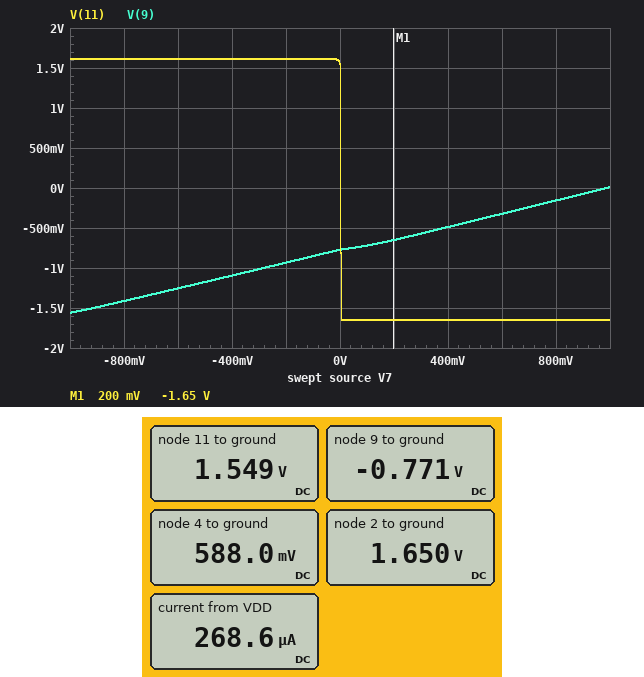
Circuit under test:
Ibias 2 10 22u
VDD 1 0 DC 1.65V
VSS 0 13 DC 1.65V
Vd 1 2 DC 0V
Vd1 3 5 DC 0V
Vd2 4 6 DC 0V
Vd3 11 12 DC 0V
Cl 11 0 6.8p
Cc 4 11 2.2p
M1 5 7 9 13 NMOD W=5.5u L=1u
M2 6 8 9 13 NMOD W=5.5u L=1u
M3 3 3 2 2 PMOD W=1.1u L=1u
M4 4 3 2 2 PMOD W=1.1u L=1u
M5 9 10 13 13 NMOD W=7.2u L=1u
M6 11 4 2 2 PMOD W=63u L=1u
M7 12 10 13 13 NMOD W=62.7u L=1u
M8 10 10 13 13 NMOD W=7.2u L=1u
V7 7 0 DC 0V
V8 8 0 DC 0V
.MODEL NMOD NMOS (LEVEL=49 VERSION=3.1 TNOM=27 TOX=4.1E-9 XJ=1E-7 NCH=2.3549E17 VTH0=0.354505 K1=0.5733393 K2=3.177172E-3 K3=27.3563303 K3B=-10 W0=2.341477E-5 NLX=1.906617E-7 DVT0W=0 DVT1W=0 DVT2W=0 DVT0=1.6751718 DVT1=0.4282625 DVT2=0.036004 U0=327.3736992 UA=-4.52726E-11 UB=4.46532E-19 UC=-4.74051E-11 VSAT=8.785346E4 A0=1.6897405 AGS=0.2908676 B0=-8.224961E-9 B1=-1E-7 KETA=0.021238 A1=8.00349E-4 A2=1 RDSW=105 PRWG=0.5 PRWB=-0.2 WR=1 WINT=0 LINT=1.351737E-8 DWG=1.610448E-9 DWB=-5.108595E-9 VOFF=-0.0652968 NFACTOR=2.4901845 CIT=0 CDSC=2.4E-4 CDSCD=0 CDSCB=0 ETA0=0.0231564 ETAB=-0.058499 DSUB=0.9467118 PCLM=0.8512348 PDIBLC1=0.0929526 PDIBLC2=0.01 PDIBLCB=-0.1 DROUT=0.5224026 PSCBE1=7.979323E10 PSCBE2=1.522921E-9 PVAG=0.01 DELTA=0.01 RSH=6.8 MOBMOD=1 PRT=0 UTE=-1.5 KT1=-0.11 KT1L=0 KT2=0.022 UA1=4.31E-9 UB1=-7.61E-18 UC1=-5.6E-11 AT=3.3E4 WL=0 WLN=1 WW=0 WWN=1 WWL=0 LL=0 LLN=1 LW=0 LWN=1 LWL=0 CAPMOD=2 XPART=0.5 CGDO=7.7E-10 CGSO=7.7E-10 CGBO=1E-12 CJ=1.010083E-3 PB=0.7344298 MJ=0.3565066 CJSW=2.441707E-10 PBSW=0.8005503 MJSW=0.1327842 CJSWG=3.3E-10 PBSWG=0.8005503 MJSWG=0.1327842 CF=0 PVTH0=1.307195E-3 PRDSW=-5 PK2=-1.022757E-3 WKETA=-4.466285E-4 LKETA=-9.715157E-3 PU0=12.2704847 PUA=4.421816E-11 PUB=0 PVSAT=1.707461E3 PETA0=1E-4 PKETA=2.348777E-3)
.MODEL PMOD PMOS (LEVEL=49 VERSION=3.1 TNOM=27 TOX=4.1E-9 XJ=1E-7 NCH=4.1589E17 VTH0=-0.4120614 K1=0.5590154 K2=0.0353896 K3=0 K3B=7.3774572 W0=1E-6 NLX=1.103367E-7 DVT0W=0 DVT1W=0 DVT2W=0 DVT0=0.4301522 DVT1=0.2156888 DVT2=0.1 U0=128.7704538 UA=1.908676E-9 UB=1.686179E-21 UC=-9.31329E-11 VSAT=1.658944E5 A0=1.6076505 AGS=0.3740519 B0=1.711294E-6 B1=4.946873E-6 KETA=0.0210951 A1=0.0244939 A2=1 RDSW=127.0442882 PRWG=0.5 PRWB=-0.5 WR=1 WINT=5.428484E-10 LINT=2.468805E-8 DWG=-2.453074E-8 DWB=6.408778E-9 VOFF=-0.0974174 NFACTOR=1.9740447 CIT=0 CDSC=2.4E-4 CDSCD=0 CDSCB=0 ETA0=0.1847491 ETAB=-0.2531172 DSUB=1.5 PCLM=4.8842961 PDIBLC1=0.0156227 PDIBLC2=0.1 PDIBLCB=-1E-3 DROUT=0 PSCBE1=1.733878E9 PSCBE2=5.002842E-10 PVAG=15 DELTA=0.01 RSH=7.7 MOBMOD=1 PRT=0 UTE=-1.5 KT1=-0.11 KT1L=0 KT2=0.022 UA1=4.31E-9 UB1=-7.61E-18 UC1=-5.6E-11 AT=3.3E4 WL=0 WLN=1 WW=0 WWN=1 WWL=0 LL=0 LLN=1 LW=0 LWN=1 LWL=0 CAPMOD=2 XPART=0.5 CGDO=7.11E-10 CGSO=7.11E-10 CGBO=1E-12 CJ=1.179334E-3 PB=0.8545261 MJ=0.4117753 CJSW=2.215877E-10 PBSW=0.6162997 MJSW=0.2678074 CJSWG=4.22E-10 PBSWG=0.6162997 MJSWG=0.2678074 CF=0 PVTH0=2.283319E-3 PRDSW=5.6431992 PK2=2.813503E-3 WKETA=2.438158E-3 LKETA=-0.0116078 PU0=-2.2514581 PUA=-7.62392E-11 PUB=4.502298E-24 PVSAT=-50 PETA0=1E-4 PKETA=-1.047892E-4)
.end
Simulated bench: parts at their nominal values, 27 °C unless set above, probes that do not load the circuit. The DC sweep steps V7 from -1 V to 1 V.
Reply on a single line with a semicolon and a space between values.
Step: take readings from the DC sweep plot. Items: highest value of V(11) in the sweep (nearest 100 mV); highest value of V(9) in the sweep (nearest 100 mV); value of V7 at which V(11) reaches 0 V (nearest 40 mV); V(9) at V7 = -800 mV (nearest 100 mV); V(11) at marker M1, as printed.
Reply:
1.6 V; 0 V; 0 V; -1.4 V; -1.65 V
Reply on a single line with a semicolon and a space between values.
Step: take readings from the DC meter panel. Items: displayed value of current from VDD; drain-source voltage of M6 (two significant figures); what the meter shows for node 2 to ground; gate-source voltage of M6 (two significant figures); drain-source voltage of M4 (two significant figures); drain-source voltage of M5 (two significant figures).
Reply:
268.6 µA; -100 mV; 1.650 V; -1.1 V; -1.1 V; 880 mV
